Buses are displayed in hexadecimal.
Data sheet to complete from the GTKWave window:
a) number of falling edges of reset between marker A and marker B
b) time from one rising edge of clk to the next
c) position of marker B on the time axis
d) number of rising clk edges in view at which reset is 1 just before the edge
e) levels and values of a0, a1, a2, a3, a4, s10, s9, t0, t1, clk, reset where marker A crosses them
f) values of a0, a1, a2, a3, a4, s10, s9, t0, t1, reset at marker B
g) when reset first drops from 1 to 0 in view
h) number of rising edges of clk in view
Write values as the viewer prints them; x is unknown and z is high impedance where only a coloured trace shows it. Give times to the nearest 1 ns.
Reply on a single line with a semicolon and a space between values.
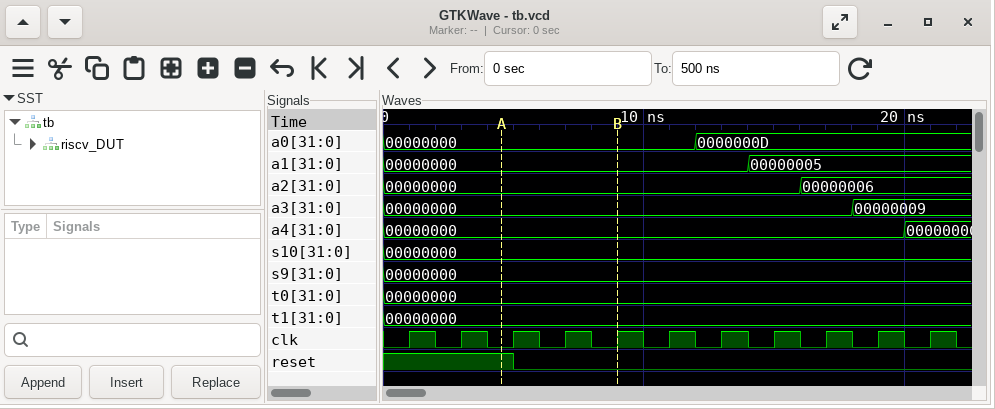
1; 2 ns; 9 ns; 3; a0=00000000, a1=00000000, a2=00000000, a3=00000000, a4=00000000, s10=00000000, s9=00000000, t0=00000000, t1=00000000, clk=0, reset=1; a0=00000000, a1=00000000, a2=00000000, a3=00000000, a4=00000000, s10=00000000, s9=00000000, t0=00000000, t1=00000000, reset=0; 5 ns; 11
